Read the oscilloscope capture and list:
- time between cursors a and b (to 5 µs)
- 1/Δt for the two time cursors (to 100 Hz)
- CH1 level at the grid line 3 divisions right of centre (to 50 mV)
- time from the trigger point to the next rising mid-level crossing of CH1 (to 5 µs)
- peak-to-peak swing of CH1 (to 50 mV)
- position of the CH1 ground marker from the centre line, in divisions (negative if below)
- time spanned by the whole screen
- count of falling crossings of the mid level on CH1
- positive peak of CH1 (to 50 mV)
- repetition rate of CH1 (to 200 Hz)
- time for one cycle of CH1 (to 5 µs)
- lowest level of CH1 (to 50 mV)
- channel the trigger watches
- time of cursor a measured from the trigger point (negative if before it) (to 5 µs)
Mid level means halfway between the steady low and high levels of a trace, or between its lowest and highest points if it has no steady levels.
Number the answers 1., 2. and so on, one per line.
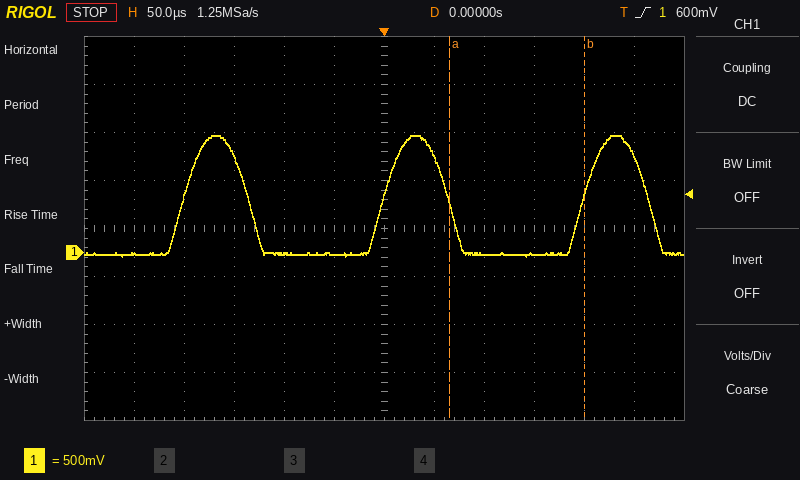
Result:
1. 135 µs
2. 7.4 kHz
3. 0 mV
4. 200 µs
5. 1.25 V
6. -0.5 div
7. 600 µs
8. 3
9. 1.20 V
10. 5.0 kHz
11. 200 µs
12. -50 mV
13. CH1
14. +65 µs
